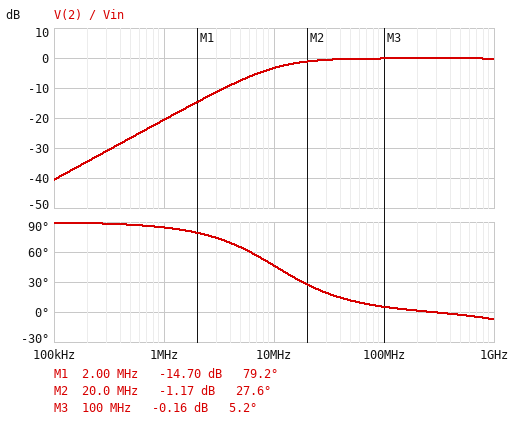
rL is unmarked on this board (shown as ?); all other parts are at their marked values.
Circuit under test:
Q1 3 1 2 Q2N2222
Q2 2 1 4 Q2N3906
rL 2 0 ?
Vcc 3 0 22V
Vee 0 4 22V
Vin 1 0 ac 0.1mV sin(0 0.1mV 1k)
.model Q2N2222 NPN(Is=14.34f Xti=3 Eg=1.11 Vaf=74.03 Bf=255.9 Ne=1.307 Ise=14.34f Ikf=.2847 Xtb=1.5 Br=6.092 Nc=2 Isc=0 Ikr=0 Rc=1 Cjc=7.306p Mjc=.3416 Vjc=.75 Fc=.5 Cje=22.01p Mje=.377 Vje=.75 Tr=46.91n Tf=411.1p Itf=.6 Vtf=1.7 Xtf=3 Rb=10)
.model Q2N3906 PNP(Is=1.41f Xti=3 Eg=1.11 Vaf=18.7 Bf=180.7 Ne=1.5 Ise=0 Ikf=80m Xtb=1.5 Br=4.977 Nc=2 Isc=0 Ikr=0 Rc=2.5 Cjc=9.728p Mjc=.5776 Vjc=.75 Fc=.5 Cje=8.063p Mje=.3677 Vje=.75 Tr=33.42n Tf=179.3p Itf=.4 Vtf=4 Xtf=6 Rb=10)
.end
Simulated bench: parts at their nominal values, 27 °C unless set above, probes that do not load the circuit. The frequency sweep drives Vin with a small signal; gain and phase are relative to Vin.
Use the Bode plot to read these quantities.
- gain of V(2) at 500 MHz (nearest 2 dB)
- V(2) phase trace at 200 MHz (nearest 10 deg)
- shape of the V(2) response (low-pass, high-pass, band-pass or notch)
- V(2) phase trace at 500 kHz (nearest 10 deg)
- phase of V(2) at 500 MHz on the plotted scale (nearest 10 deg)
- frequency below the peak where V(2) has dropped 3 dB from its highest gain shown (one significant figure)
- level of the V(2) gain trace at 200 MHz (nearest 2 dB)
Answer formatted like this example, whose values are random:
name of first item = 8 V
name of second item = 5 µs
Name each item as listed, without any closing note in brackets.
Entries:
gain of V(2) at 500 MHz = 0 dB
V(2) phase trace at 200 MHz = 0 deg
shape of the V(2) response = high-pass
V(2) phase trace at 500 kHz = 90 deg
phase of V(2) at 500 MHz on the plotted scale = 0 deg
frequency below the peak where V(2) has dropped 3 dB from its highest gain shown = 10 MHz
level of the V(2) gain trace at 200 MHz = 0 dB
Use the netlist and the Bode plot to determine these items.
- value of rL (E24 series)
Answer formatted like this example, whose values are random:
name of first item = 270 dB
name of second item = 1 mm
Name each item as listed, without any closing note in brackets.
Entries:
value of rL = 470 Ω
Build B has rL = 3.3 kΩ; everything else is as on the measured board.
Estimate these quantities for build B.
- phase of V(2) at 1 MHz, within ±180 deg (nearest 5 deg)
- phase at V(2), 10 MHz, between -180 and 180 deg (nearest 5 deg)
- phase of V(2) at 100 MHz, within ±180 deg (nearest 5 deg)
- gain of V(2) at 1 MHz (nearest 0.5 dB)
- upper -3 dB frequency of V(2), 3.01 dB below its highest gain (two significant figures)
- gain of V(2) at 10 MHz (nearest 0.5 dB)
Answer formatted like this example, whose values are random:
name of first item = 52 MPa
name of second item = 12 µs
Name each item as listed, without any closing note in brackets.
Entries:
phase of V(2) at 1 MHz, within ±180 deg = 55 deg
phase at V(2), 10 MHz, between -180 and 180 deg = 10 deg
phase of V(2) at 100 MHz, within ±180 deg = 0 deg
gain of V(2) at 1 MHz = -5.0 dB
upper -3 dB frequency of V(2), 3.01 dB below its highest gain = 6.6 GHz
gain of V(2) at 10 MHz = 0 dB
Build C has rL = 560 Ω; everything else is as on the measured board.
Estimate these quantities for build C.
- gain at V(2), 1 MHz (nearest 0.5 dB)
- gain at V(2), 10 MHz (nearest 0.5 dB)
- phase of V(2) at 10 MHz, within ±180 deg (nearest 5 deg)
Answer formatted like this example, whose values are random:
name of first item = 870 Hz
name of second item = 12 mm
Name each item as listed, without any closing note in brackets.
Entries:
gain at V(2), 1 MHz = -19.0 dB
gain at V(2), 10 MHz = -2.5 dB
phase of V(2) at 10 MHz, within ±180 deg = 40 deg
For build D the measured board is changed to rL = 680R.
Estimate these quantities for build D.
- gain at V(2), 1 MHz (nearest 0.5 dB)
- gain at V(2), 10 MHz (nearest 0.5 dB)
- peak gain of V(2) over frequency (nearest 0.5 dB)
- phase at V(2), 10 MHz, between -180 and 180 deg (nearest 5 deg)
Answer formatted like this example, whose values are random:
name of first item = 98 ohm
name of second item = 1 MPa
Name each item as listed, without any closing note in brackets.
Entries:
gain at V(2), 1 MHz = -17.5 dB
gain at V(2), 10 MHz = -2.0 dB
peak gain of V(2) over frequency = 0 dB
phase at V(2), 10 MHz, between -180 and 180 deg = 35 deg
